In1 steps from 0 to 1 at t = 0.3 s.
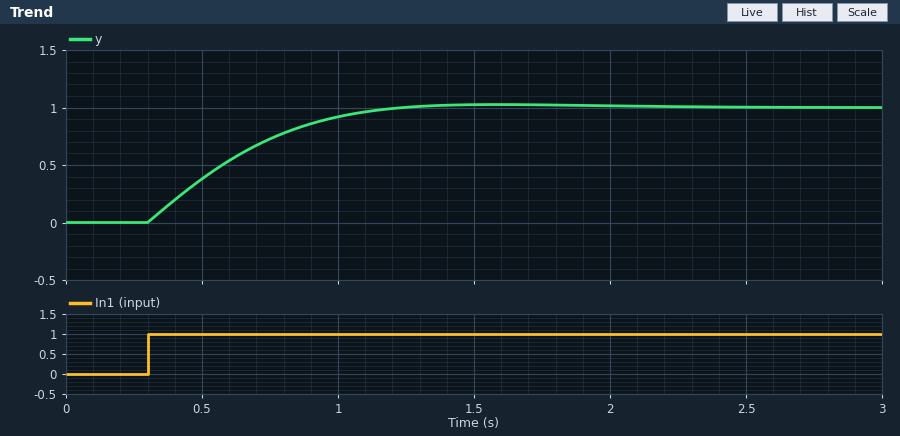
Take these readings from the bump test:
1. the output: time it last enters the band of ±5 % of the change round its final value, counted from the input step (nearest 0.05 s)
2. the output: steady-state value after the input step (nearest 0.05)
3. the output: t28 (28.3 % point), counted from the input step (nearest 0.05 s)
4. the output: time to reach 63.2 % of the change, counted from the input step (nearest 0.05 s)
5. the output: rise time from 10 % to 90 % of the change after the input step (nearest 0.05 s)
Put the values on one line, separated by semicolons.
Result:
0.75 s; 1.00; 0.15 s; 0.35 s; 0.60 s
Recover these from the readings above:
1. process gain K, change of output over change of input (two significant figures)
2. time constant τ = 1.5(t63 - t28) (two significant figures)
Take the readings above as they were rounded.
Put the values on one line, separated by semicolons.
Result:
1.0; 0.30 s
